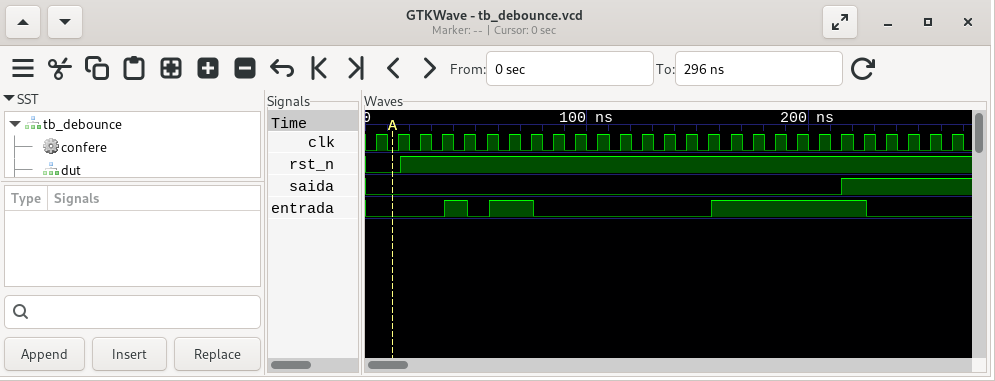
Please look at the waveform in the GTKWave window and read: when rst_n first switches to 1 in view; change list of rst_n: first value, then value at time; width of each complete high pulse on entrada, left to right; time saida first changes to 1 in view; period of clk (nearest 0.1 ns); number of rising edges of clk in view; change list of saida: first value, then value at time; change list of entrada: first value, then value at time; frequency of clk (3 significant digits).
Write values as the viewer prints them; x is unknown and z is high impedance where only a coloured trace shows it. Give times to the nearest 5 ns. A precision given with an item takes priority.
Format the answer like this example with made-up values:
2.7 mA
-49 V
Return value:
15 ns
0, 1 at 15 ns
10 ns, 20 ns, 70 ns
215 ns
10 ns
27
0, 1 at 215 ns
0, 1 at 35 ns, 0 at 45 ns, 1 at 55 ns, 0 at 75 ns, 1 at 155 ns, 0 at 225 ns
100 MHz
